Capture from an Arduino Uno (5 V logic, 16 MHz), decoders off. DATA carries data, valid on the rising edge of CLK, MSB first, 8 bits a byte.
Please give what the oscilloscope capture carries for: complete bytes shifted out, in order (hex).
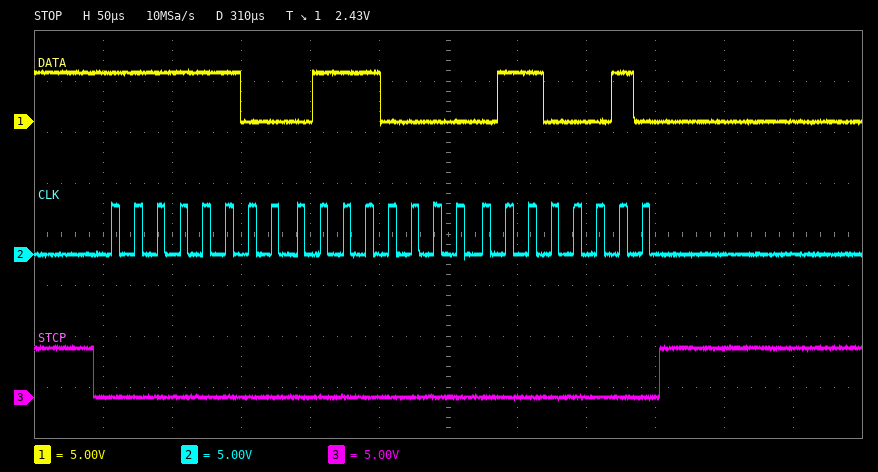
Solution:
FC 70 62
